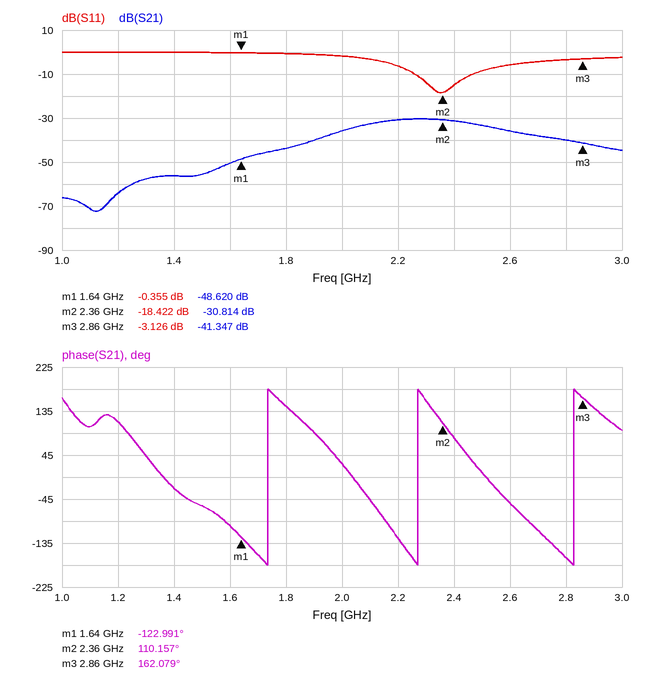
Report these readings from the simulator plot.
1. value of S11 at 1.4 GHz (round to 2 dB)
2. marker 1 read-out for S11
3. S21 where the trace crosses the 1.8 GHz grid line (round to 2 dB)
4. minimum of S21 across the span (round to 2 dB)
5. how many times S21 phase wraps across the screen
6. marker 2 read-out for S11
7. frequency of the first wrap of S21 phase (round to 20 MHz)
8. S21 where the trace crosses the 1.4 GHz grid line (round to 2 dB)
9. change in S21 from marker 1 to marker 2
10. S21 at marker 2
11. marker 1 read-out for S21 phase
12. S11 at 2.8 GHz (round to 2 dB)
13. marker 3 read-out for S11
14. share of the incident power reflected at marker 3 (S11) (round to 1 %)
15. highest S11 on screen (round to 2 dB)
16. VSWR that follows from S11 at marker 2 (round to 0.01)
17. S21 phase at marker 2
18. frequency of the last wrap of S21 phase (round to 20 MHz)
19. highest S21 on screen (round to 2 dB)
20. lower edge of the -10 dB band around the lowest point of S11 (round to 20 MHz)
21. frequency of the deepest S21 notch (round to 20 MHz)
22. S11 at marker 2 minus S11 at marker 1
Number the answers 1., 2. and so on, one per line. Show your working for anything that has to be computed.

1. 0 dB
2. -0.355 dB
3. -44 dB
4. -72 dB
5. 3
6. -18.422 dB
7. 1.74 GHz
8. -56 dB
9. -30.814 − (-48.62) = 17.806 dB
10. -30.814 dB
11. -122.991°
12. -4 dB
13. -3.126 dB
14. 10^(-3.126/10) ≈ 49 %
15. 0 dB
16. (1 + 0.1199)/(1 − 0.1199) ≈ 1.27
17. 110.157°
18. 2.82 GHz
19. -30 dB
20. 2.26 GHz
21. 1.12 GHz
22. -18.422 − (-0.355) = -18.067 dB
